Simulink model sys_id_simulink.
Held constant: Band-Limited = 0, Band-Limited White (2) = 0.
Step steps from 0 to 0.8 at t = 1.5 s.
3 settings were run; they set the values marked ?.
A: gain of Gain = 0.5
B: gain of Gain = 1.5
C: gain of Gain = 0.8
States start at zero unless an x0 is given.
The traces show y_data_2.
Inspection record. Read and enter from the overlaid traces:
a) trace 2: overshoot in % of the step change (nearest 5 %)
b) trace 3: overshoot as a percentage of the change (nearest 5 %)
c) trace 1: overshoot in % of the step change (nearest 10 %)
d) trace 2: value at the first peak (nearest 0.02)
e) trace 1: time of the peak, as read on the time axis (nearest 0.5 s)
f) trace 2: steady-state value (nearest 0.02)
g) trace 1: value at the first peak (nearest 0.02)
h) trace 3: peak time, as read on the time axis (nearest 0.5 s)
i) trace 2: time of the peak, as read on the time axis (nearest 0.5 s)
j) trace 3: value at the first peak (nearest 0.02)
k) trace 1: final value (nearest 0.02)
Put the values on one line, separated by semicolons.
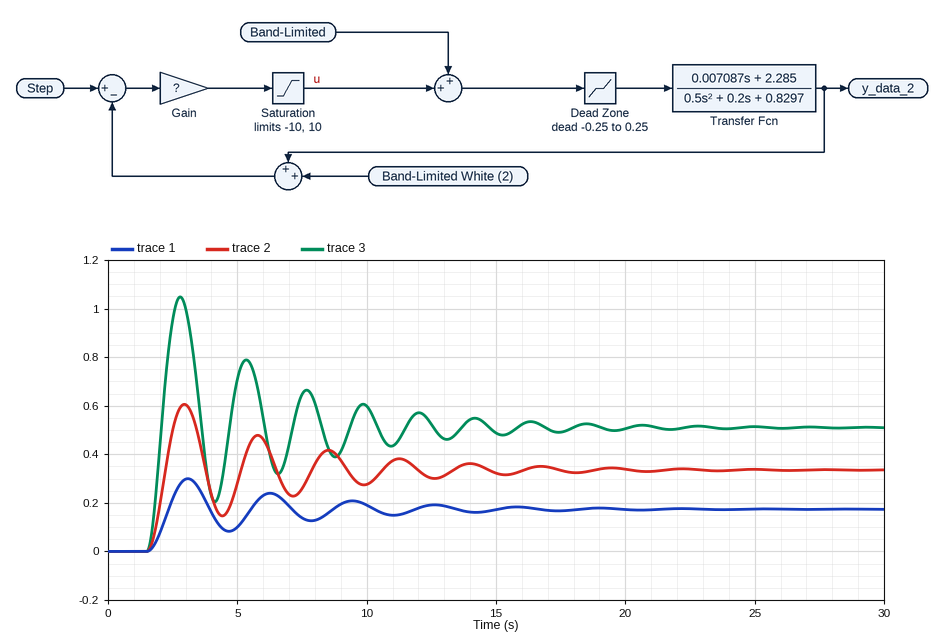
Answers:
80 %; 105 %; 70 %; 0.60; 3.0 s; 0.34; 0.30; 3.0 s; 3.0 s; 1.04; 0.18
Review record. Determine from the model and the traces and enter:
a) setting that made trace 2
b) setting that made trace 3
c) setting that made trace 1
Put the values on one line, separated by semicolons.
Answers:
C; B; A
